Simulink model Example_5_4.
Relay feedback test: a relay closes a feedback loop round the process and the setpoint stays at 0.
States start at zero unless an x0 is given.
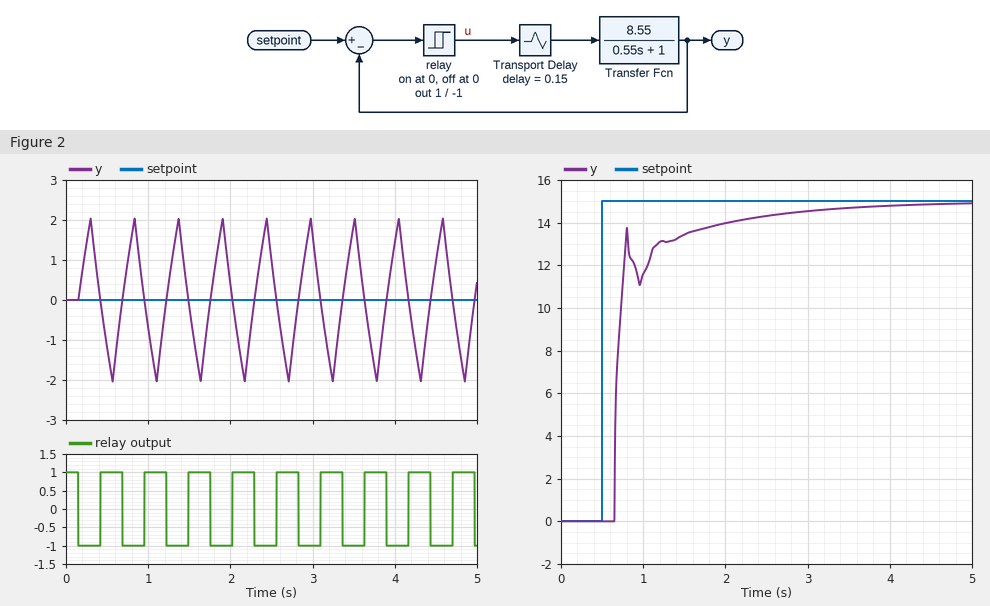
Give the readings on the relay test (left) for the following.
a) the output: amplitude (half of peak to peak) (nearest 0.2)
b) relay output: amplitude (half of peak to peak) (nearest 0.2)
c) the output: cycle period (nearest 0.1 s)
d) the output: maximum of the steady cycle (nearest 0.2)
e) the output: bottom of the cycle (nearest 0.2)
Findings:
2.0
1.0
0.5 s
2.0
-2.0
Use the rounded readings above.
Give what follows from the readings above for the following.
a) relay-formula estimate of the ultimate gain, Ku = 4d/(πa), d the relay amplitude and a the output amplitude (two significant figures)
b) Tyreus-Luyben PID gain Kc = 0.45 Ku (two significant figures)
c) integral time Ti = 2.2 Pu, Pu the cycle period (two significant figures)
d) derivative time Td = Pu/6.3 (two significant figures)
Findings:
0.64
0.29
1.1 s
0.079 s
